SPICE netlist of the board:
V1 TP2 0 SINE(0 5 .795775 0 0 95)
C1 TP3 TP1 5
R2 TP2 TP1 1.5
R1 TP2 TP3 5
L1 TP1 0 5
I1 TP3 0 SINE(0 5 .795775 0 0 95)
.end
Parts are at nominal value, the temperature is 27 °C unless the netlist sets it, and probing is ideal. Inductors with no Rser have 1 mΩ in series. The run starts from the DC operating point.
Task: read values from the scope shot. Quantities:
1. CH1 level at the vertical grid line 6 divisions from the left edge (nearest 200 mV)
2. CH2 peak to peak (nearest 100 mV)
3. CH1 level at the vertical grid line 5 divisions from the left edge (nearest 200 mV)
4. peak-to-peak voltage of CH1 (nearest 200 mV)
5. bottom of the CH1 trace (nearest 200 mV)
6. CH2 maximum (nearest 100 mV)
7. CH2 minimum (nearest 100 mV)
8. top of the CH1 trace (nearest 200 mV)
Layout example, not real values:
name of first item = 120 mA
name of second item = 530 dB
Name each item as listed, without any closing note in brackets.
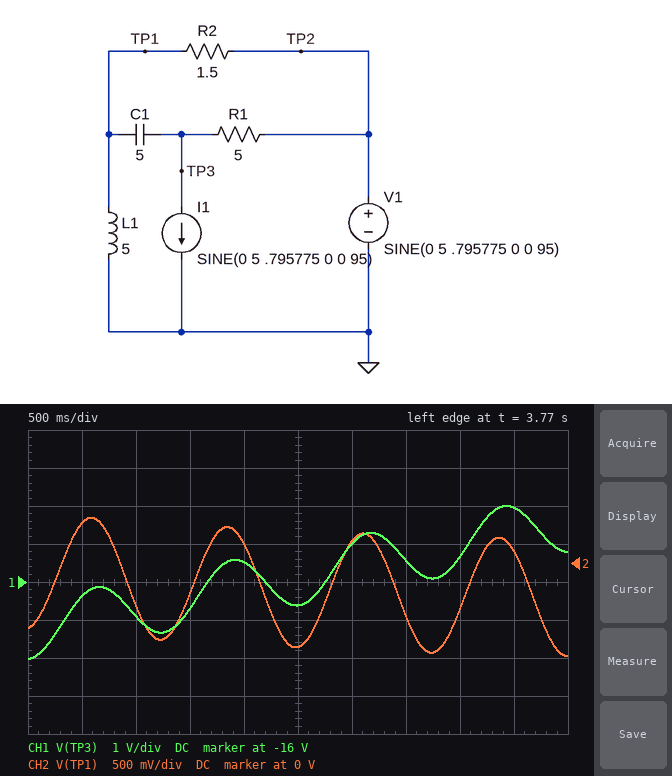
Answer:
CH1 level at the vertical grid line 6 divisions from the left edge = -15.0 V
CH2 peak to peak = 1.8 V
CH1 level at the vertical grid line 5 divisions from the left edge = -16.6 V
peak-to-peak voltage of CH1 = 4.0 V
bottom of the CH1 trace = -18.0 V
CH2 maximum = 600 mV
CH2 minimum = -1.2 V
top of the CH1 trace = -14.0 V
